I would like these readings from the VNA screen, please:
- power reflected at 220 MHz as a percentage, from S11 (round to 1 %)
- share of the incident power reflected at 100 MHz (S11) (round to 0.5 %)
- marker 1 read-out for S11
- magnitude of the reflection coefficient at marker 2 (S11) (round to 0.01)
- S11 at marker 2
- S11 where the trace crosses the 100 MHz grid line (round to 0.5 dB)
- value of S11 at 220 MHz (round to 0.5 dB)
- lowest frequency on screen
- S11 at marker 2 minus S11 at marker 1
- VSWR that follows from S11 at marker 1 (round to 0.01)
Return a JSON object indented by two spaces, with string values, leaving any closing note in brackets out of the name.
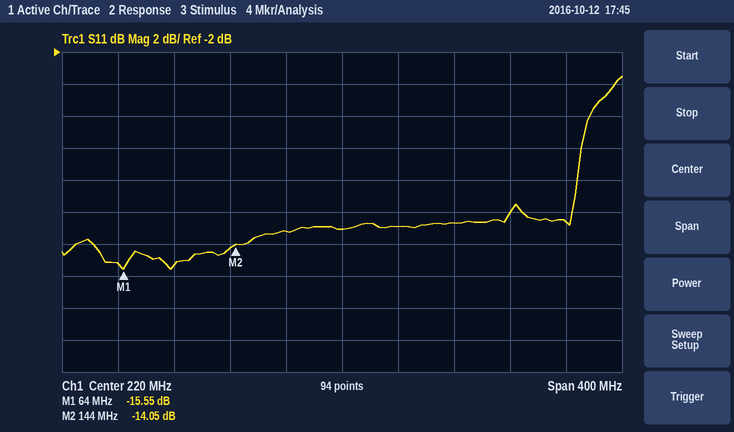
{
  "power reflected at 220 MHz as a percentage, from S11": "5 %",
  "share of the incident power reflected at 100 MHz (S11)": "3.0 %",
  "marker 1 read-out for S11": "-15.55 dB",
  "magnitude of the reflection coefficient at marker 2 (S11)": "0.20",
  "S11 at marker 2": "-14.05 dB",
  "S11 where the trace crosses the 100 MHz grid line": "-15.5 dB",
  "value of S11 at 220 MHz": "-13.0 dB",
  "lowest frequency on screen": "20 MHz",
  "S11 at marker 2 minus S11 at marker 1": "1.50 dB",
  "VSWR that follows from S11 at marker 1": "1.40"
}
